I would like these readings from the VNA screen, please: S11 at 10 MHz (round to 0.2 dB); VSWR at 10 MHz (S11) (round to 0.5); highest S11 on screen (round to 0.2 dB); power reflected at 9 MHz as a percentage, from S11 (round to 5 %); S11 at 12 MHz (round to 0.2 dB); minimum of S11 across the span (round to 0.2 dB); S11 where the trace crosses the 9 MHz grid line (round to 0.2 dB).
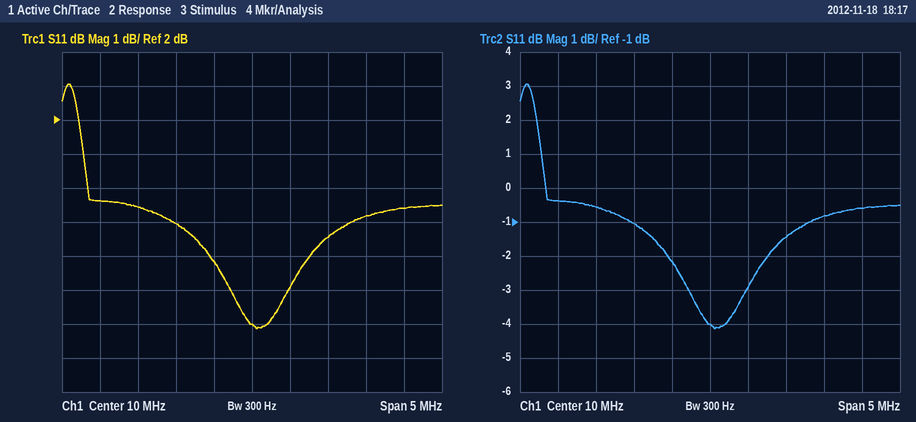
-4.0 dB
4.5
3.0 dB
80 %
-0.6 dB
-4.2 dB
-1.0 dB
